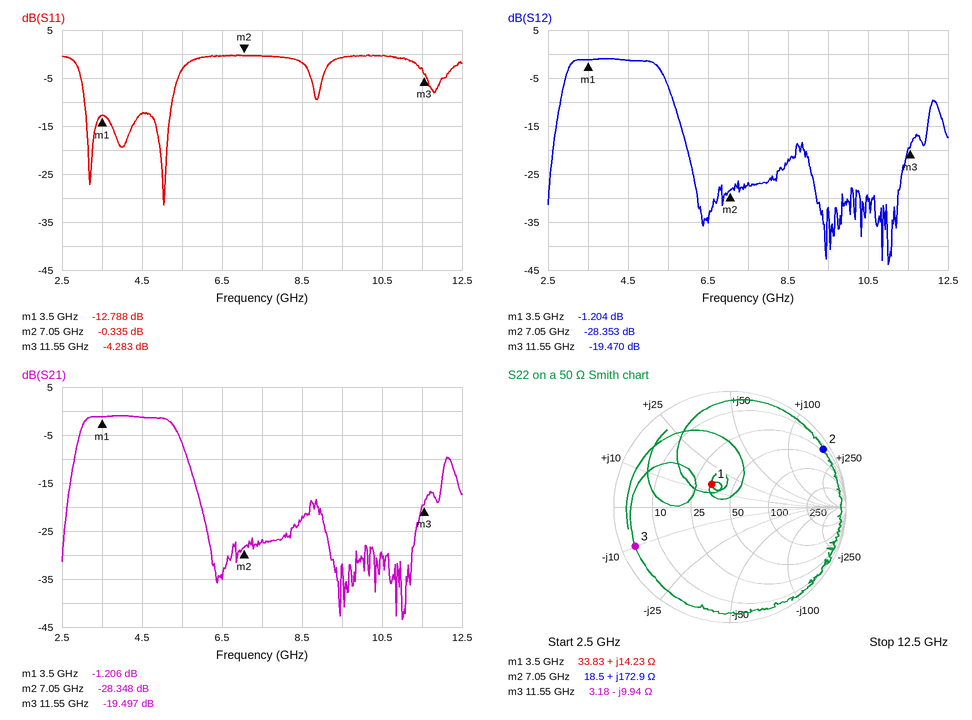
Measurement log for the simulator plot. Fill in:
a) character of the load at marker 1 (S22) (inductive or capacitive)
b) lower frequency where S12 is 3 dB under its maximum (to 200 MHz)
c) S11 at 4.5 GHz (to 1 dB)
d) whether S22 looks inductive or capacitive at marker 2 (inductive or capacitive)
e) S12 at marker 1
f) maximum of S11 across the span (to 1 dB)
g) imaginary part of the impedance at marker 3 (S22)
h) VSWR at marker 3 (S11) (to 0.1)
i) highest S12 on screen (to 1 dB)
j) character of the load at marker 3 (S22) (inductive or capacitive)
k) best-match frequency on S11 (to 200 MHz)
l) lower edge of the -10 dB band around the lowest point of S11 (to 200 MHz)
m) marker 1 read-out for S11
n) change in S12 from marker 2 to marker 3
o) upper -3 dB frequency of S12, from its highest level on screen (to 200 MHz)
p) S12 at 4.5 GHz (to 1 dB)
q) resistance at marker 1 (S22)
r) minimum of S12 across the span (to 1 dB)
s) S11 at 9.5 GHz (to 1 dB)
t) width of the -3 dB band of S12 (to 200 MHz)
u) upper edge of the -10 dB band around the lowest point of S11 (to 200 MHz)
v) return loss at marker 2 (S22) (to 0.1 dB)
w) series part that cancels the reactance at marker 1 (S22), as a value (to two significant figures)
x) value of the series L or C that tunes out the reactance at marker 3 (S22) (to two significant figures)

inductive
3.0 GHz
-12 dB
inductive
-1.204 dB
0 dB
-9.94 Ω
4.1
-1 dB
capacitive
5.0 GHz
3.0 GHz
-12.788 dB
8.883 dB
5.4 GHz
-1 dB
33.83 Ω
-44 dB
-1 dB
2.4 GHz
5.2 GHz
0.5 dB
3.2 pF
140 pH
